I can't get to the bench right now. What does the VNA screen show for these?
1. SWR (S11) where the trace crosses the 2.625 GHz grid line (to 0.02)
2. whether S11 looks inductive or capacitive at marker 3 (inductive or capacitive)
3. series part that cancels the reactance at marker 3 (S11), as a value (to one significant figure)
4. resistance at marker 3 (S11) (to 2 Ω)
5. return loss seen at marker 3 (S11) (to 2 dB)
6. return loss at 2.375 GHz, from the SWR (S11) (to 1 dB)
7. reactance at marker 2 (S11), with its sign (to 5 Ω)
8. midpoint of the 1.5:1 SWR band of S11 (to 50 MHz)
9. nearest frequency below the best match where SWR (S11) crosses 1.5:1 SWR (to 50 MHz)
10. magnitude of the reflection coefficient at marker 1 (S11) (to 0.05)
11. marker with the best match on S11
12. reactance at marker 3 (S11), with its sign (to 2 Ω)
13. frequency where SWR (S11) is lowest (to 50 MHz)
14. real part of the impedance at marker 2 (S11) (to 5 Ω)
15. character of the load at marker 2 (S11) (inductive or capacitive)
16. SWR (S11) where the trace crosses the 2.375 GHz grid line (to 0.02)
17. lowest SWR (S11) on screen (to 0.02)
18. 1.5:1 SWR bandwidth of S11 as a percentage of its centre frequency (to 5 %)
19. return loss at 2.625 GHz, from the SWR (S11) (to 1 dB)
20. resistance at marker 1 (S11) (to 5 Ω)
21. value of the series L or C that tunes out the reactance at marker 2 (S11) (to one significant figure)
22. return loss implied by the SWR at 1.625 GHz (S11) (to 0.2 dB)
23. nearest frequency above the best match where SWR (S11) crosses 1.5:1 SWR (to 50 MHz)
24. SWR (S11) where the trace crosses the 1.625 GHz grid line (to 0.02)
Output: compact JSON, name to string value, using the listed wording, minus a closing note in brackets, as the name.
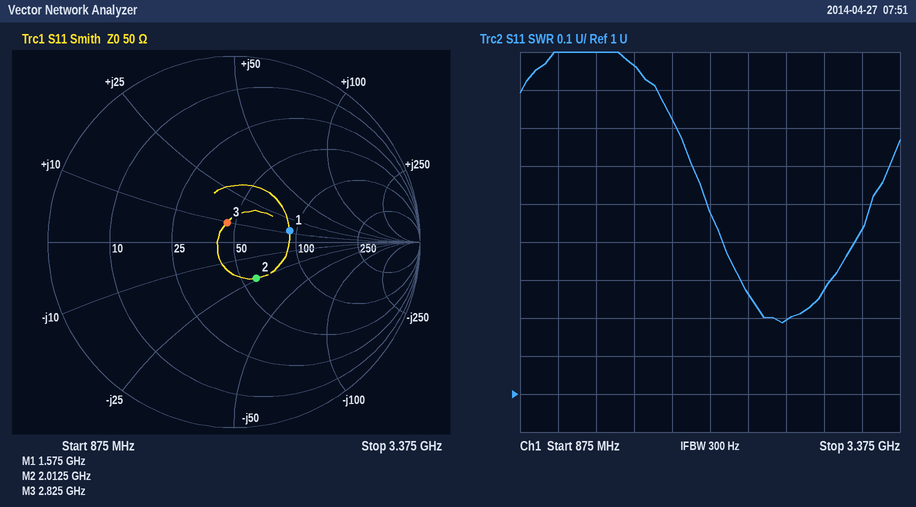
{"SWR (S11) where the trace crosses the 2.625 GHz grid line": "1.20", "whether S11 looks inductive or capacitive at marker 3": "inductive", "series part that cancels the reactance at marker 3 (S11), as a value": "6 pF", "resistance at marker 3 (S11)": "46 Ω", "return loss seen at marker 3 (S11)": "20 dB", "return loss at 2.375 GHz, from the SWR (S11)": "19 dB", "reactance at marker 2 (S11), with its sign": "-25 Ω", "midpoint of the 1.5:1 SWR band of S11": "2.65 GHz", "nearest frequency below the best match where SWR (S11) crosses 1.5:1 SWR": "2.10 GHz", "magnitude of the reflection coefficient at marker 1 (S11)": "0.30", "marker with the best match on S11": "marker 3", "reactance at marker 3 (S11), with its sign": "+10 Ω", "frequency where SWR (S11) is lowest": "2.60 GHz", "real part of the impedance at marker 2 (S11)": "60 Ω", "character of the load at marker 2 (S11)": "capacitive", "SWR (S11) where the trace crosses the 2.375 GHz grid line": "1.26", "lowest SWR (S11) on screen": "1.18", "1.5:1 SWR bandwidth of S11 as a percentage of its centre frequency": "40 %", "return loss at 2.625 GHz, from the SWR (S11)": "21 dB", "resistance at marker 1 (S11)": "90 Ω", "value of the series L or C that tunes out the reactance at marker 2 (S11)": "2 nH", "return loss implied by the SWR at 1.625 GHz (S11)": "10.4 dB", "nearest frequency above the best match where SWR (S11) crosses 1.5:1 SWR": "3.20 GHz", "SWR (S11) where the trace crosses the 1.625 GHz grid line": "1.86"}
